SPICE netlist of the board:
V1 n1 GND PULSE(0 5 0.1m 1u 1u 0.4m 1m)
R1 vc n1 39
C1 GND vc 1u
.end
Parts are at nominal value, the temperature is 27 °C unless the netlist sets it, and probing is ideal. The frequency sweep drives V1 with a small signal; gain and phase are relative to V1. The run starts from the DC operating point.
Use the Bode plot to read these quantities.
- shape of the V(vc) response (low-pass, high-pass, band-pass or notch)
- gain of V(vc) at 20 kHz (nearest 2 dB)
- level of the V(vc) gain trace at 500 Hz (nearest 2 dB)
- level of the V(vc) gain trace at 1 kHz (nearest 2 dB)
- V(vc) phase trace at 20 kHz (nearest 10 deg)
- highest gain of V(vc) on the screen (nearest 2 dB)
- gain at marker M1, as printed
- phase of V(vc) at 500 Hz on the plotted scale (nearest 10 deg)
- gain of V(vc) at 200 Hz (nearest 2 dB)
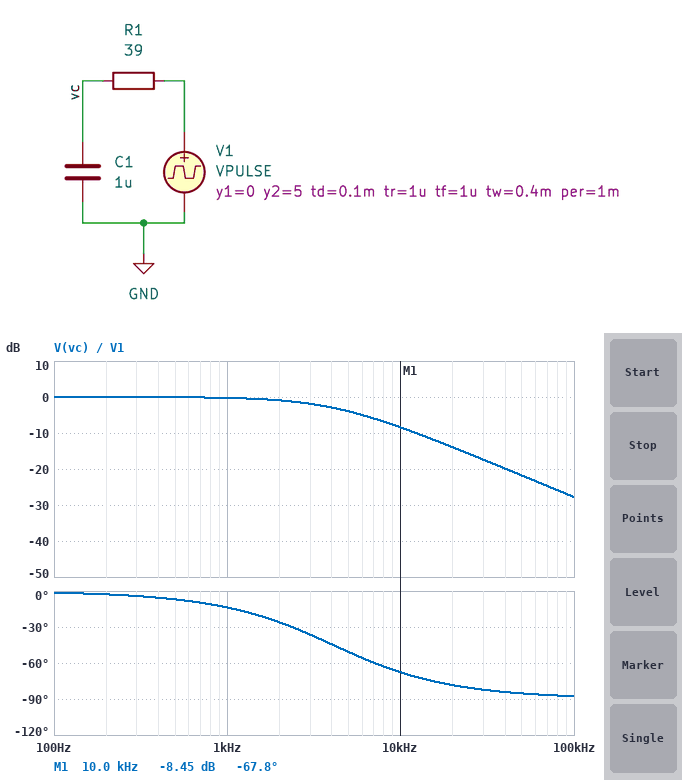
low-pass
-14 dB
0 dB
0 dB
-80 deg
0 dB
-8.45 dB
-10 deg
0 dB
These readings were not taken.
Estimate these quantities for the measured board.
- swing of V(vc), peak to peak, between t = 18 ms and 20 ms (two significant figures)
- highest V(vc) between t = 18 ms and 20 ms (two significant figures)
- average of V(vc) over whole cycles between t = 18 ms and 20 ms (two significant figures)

5.0 V
5.0 V
2.0 V
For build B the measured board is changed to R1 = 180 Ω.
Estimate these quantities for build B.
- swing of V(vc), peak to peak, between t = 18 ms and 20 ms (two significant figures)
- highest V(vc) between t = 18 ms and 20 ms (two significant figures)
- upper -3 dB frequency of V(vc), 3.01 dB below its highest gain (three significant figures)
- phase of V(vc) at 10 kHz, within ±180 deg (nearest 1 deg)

4.3 V
4.5 V
884 Hz
-85 deg
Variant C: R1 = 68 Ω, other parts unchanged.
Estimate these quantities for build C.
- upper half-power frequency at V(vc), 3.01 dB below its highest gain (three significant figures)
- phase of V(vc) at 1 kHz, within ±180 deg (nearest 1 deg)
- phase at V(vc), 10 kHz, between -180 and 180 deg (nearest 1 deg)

2.34 kHz
-23 deg
-77 deg
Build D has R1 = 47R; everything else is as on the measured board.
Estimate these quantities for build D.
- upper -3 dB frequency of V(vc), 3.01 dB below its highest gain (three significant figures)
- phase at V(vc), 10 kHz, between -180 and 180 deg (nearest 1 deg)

3.39 kHz
-71 deg
